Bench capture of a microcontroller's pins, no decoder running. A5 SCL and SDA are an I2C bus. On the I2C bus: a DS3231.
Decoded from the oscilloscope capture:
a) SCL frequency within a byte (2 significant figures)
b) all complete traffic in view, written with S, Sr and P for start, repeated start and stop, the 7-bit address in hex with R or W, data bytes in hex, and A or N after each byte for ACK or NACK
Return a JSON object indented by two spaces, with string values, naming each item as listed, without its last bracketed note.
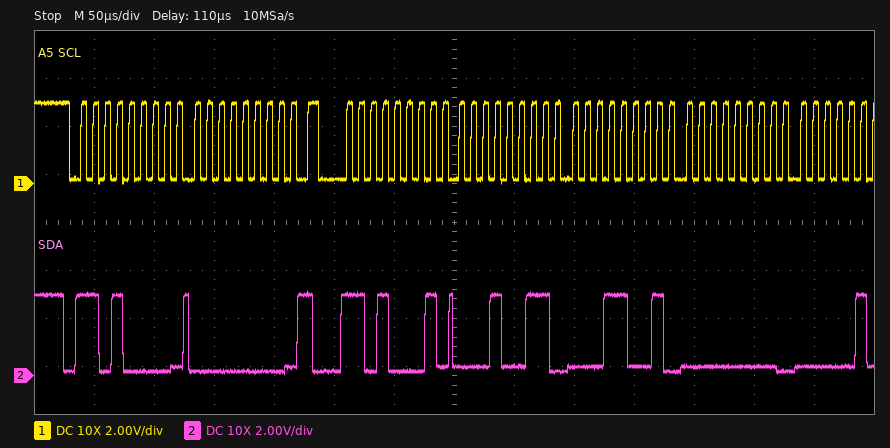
{
  "SCL frequency within a byte": "100 kHz",
  "all complete traffic in view, written with S, Sr and P for start, repeated start and stop, the 7-bit address in hex with R or W, data bytes in hex, and A or N after each byte for ACK or NACK": "S 68W A 00 A Sr 68R A 13 A 19 A 00 A"
}
